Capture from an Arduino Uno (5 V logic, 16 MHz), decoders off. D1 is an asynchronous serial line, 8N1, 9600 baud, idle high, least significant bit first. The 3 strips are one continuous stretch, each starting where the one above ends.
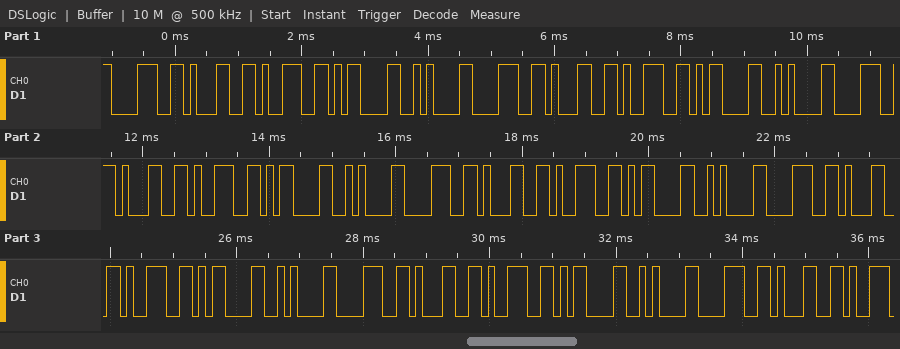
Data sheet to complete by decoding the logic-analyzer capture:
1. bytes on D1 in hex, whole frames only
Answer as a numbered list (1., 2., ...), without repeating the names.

1. 0x38 0x31 0x39 0x0D 0x0A 0x38 0x31 0x39 0x0D 0x0A 0x38 0x31 0x39 0x0D 0x0A 0x38 0x31 0x39 0x0D 0x0A 0x38 0x31 0x39 0x0D 0x0A 0x38 0x31 0x39 0x0D 0x0A 0x38 0x31
